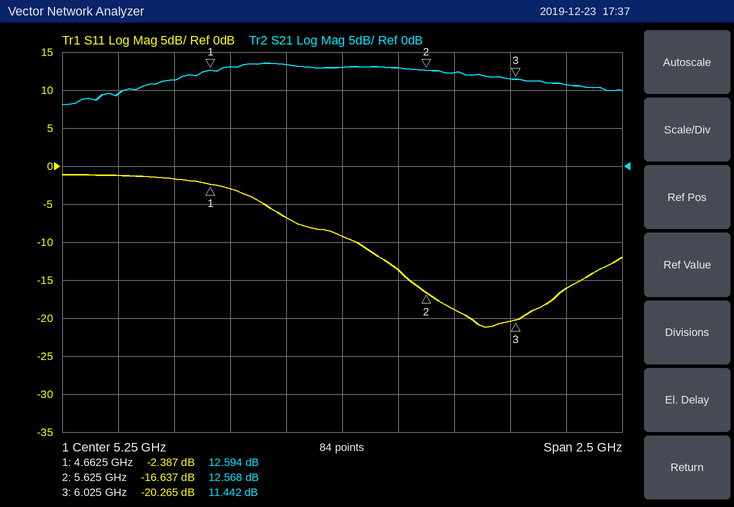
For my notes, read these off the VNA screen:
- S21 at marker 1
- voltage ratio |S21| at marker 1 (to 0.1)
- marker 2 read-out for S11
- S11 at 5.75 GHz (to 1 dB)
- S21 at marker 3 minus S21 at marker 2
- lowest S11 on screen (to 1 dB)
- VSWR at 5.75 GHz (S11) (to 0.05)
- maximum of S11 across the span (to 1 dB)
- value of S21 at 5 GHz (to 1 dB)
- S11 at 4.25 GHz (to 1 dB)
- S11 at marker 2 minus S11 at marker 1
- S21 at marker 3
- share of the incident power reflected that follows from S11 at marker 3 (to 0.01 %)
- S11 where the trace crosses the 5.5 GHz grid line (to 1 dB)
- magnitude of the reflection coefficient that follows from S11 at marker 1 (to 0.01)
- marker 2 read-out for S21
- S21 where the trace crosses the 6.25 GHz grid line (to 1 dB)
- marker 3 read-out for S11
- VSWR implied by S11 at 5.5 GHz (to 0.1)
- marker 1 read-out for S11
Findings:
12.594 dB
4.3
-16.637 dB
-19 dB
-1.126 dB
-21 dB
1.25
-1 dB
13 dB
-1 dB
-14.250 dB
11.442 dB
0.94 %
-14 dB
0.76
12.568 dB
11 dB
-20.265 dB
1.5
-2.387 dB
